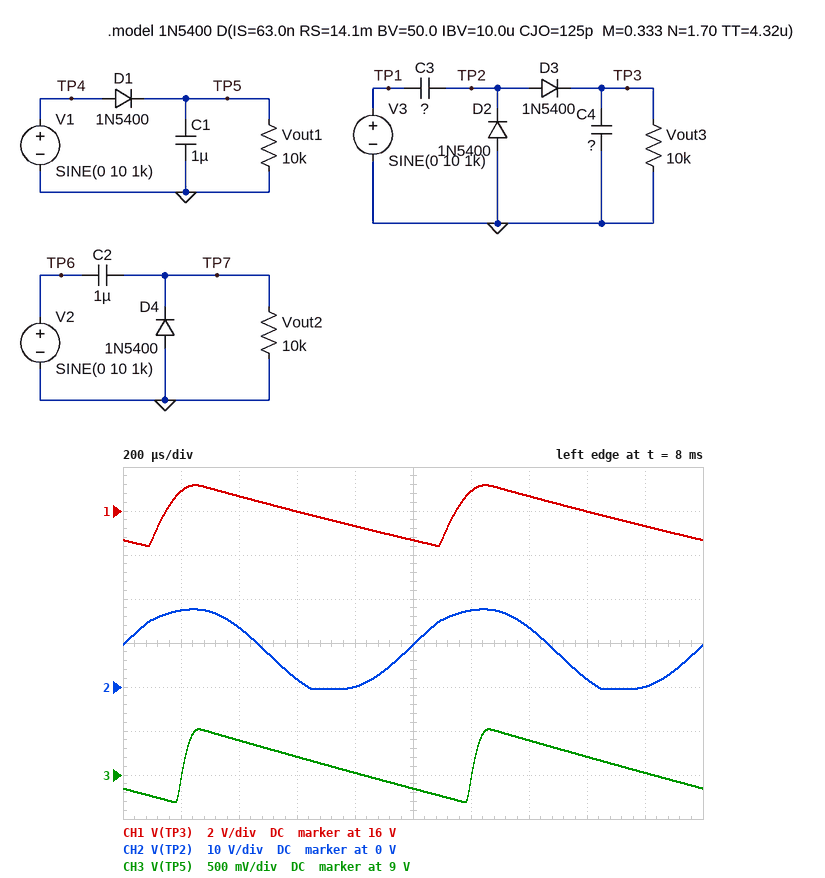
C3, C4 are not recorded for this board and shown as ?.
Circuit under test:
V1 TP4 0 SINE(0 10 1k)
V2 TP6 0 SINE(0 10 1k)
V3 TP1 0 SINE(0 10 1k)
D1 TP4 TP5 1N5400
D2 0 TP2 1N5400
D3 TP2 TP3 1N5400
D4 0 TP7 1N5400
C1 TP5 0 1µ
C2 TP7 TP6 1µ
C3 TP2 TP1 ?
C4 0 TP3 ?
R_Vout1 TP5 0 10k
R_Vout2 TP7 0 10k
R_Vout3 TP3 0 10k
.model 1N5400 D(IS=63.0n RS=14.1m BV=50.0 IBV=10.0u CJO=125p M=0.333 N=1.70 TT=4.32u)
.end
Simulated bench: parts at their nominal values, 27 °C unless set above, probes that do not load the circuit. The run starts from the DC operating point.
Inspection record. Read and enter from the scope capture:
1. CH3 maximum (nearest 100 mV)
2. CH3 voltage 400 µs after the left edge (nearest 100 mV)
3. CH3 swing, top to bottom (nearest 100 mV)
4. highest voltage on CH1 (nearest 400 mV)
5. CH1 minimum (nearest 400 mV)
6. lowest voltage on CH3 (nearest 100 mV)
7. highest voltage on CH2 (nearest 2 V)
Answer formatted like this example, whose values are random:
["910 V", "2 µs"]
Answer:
["9.5 V", "9.4 V", "800 mV", "17.2 V", "14.4 V", "8.7 V", "18 V"]
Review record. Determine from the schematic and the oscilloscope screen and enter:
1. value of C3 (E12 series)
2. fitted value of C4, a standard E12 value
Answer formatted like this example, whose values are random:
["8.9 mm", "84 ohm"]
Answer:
["820 nF", "470 nF"]
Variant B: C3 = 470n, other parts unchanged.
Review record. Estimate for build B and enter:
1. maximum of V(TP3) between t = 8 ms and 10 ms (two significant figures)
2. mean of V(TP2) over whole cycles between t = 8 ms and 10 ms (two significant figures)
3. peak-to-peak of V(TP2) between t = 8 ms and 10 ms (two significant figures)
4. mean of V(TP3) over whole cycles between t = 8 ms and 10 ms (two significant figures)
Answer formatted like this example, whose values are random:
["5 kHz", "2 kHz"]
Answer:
["16 V", "7.9 V", "17 V", "15 V"]
